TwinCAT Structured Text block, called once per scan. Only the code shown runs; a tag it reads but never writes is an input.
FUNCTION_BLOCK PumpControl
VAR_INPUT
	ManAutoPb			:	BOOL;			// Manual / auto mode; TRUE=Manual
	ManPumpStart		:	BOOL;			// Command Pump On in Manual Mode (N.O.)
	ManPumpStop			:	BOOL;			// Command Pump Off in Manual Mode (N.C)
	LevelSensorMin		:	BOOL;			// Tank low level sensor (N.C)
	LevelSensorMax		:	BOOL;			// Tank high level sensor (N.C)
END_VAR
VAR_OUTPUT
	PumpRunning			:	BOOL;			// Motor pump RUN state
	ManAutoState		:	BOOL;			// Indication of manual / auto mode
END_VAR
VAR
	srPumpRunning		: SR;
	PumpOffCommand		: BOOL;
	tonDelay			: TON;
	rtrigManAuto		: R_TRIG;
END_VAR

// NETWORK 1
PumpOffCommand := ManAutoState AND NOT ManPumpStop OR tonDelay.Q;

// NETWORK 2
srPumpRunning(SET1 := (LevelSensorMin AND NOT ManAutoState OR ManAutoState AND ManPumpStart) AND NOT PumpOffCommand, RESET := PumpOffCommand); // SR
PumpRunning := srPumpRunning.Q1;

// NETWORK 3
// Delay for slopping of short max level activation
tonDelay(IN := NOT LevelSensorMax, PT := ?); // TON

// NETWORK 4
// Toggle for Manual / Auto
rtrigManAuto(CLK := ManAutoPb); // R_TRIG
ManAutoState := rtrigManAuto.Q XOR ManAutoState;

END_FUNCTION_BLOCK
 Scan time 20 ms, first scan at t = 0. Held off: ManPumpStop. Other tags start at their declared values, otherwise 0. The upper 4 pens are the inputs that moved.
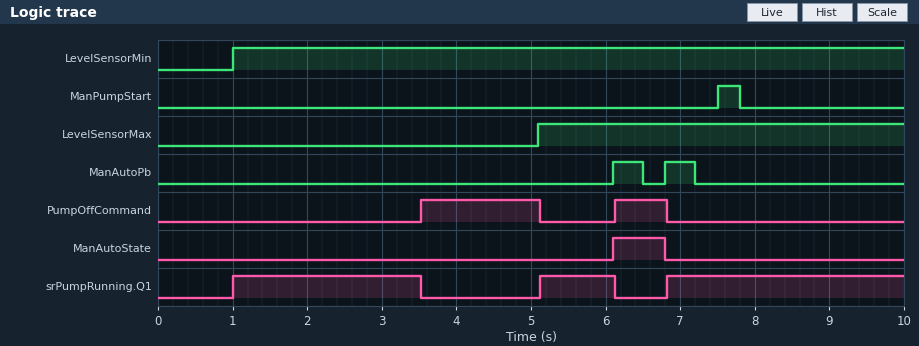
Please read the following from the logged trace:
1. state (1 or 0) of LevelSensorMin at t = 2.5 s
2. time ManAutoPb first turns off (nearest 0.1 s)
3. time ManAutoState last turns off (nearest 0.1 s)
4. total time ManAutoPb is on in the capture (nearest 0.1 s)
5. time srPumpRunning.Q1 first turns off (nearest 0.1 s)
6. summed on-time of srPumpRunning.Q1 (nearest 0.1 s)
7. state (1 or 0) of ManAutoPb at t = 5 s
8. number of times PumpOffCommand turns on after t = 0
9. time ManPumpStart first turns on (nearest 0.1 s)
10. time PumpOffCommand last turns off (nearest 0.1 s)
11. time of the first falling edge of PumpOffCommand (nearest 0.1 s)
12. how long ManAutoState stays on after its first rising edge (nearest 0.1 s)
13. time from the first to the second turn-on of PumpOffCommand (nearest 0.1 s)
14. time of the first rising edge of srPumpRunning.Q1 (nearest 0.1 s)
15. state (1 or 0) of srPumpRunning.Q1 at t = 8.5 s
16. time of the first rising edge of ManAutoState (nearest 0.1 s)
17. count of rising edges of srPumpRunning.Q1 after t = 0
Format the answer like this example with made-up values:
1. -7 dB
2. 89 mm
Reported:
1. 1
2. 6.5 s
3. 6.8 s
4. 0.8 s
5. 3.5 s
6. 6.7 s
7. 0
8. 2
9. 7.5 s
10. 6.8 s
11. 5.1 s
12. 0.7 s
13. 2.6 s
14. 1.0 s
15. 1
16. 6.1 s
17. 3
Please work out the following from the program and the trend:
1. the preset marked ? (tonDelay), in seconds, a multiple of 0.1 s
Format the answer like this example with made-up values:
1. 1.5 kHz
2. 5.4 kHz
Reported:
1. 3.5 s
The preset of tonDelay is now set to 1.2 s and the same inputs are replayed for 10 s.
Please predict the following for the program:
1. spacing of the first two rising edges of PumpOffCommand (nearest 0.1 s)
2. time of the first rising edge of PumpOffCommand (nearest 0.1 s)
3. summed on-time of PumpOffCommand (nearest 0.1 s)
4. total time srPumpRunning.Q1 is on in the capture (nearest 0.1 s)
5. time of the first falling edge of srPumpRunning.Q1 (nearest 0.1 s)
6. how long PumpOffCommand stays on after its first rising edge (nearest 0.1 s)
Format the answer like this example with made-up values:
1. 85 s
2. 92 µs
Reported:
1. 4.9 s
2. 1.2 s
3. 4.6 s
4. 4.4 s
5. 1.2 s
6. 3.9 s
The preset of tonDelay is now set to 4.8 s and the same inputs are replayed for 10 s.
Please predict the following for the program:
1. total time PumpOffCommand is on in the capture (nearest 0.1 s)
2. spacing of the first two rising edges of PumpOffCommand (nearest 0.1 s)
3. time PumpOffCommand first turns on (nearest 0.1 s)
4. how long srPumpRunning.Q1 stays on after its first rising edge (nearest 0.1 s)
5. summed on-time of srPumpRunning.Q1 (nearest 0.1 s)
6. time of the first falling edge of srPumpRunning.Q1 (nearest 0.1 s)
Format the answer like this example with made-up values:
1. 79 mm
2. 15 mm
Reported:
1. 1.0 s
2. 1.3 s
3. 4.8 s
4. 3.8 s
5. 8.0 s
6. 4.8 s
